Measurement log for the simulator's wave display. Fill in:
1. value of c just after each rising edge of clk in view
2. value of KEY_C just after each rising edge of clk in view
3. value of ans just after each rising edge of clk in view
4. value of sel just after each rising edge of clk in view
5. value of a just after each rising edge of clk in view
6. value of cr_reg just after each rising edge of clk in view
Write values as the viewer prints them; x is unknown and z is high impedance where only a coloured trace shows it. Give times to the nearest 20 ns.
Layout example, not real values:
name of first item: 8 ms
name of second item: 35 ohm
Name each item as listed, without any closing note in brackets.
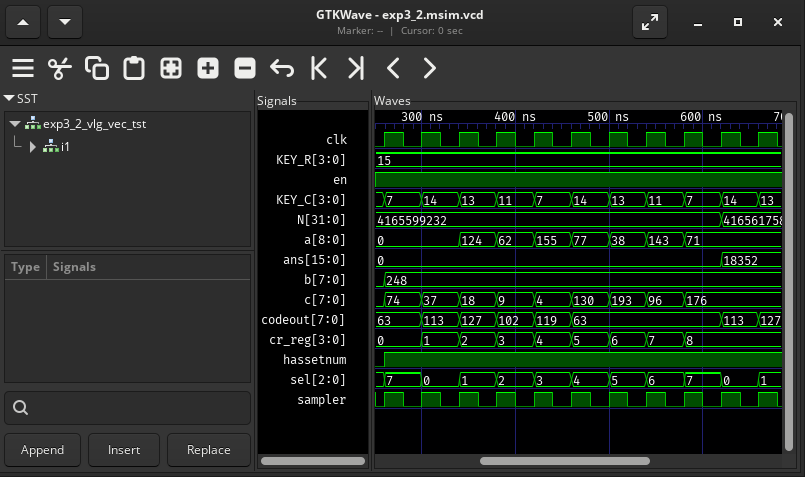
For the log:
value of c just after each rising edge of clk in view: 74, 37, 18, 9, 4, 130, 193, 96, 176, 176, 176
value of KEY_C just after each rising edge of clk in view: 7, 14, 13, 11, 7, 14, 13, 11, 7, 14, 13
value of ans just after each rising edge of clk in view: 0, 0, 0, 0, 0, 0, 0, 0, 0, 18352, 18352
value of sel just after each rising edge of clk in view: 7, 0, 1, 2, 3, 4, 5, 6, 7, 0, 1
value of a just after each rising edge of clk in view: 0, 0, 124, 62, 155, 77, 38, 143, 71, 71, 71
value of cr_reg just after each rising edge of clk in view: 0, 1, 2, 3, 4, 5, 6, 7, 8, 8, 8
